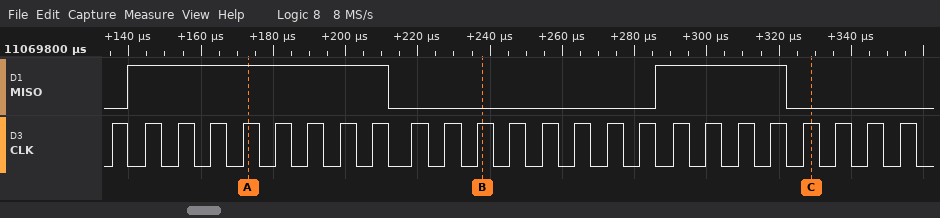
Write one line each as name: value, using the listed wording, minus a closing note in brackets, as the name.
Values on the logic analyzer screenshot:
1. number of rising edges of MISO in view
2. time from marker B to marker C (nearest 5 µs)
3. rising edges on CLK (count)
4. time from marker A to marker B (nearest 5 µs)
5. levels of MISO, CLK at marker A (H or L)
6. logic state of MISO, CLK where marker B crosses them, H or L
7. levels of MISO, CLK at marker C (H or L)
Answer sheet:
number of rising edges of MISO in view: 2
time from marker B to marker C: 90 µs
rising edges on CLK: 25
time from marker A to marker B: 65 µs
levels of MISO, CLK at marker A: MISO=H, CLK=H
logic state of MISO, CLK where marker B crosses them, H or L: MISO=L, CLK=H
levels of MISO, CLK at marker C: MISO=L, CLK=H
